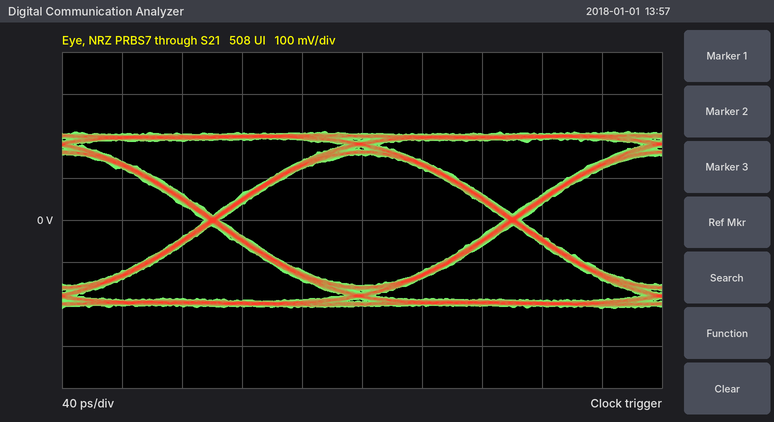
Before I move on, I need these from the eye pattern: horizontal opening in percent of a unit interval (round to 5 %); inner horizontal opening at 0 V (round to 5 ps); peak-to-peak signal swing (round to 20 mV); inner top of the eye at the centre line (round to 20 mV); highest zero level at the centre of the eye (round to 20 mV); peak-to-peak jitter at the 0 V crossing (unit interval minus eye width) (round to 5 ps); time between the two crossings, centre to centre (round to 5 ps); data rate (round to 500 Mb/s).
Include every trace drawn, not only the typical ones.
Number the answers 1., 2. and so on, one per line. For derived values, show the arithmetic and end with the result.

1. 190 ps / 200 ps ≈ 95 %
2. 190 ps
3. 420 mV
4. 160 mV
5. -160 mV
6. 10 ps
7. 200 ps
8. 5.0 Gb/s
